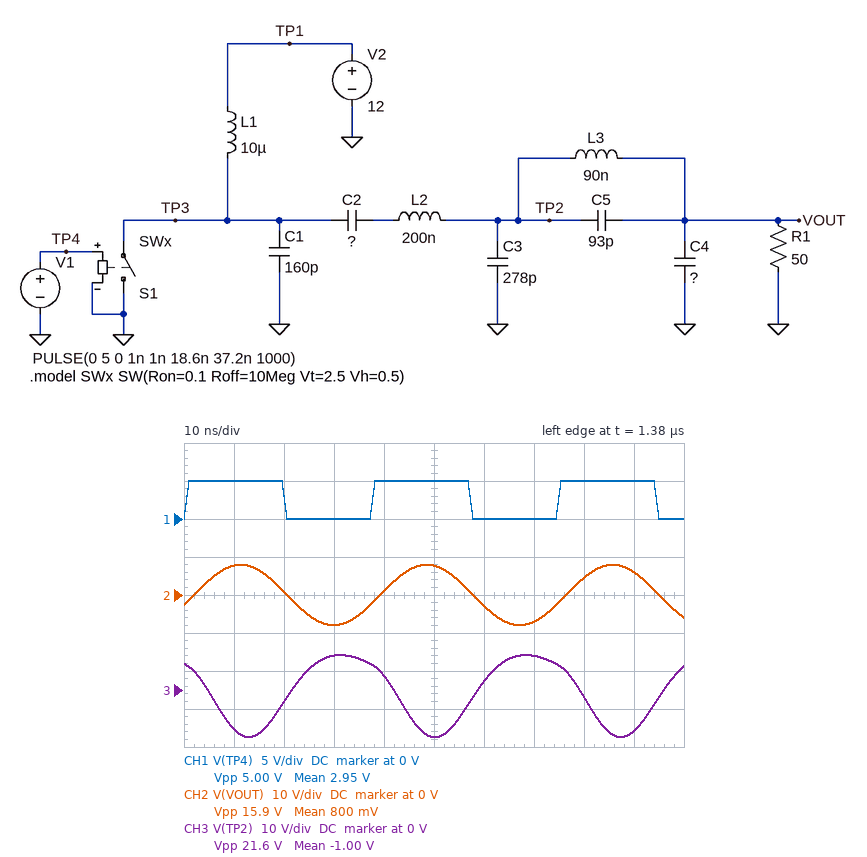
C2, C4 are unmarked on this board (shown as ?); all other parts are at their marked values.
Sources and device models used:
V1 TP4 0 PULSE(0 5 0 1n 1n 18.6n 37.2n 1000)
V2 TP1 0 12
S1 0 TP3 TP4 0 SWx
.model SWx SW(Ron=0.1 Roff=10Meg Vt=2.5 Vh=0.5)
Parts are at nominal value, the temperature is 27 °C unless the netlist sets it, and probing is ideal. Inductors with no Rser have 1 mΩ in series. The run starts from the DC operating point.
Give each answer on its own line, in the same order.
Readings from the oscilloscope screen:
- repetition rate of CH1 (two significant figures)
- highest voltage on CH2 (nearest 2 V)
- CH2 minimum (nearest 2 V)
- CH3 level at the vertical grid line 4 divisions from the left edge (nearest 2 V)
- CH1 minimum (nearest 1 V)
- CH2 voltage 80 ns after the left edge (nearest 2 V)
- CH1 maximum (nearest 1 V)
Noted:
27 MHz
8 V
-8 V
4 V
0 V
4 V
5 V
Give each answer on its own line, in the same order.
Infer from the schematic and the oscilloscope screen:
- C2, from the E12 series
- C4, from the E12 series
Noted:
390 pF
680 pF
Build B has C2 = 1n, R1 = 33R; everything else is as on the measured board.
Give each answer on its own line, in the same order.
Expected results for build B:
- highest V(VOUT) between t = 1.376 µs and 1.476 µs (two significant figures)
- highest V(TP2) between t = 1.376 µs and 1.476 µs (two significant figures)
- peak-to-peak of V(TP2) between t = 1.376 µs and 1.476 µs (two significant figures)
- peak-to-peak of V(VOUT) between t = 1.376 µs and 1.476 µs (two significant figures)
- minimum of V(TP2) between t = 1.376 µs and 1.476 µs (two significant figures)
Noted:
6.5 V
7.7 V
18 V
13 V
-11 V
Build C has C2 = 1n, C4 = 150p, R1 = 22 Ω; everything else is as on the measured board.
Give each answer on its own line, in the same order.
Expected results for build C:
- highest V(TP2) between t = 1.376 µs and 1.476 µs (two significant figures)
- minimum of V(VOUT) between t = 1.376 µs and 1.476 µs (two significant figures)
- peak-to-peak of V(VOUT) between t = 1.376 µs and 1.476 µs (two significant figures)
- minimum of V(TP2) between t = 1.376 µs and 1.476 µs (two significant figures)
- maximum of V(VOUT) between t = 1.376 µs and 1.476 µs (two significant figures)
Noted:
15 V
-14 V
27 V
-13 V
14 V
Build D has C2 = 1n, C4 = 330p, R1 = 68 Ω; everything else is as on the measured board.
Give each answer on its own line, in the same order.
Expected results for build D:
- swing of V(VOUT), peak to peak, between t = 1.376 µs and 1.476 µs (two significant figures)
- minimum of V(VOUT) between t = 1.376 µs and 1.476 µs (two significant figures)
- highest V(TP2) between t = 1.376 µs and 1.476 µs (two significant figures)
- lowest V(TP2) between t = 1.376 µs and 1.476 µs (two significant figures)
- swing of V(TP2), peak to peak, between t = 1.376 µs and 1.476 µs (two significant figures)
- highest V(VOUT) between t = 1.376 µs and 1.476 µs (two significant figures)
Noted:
24 V
-12 V
5.0 V
-4.2 V
9.2 V
12 V
